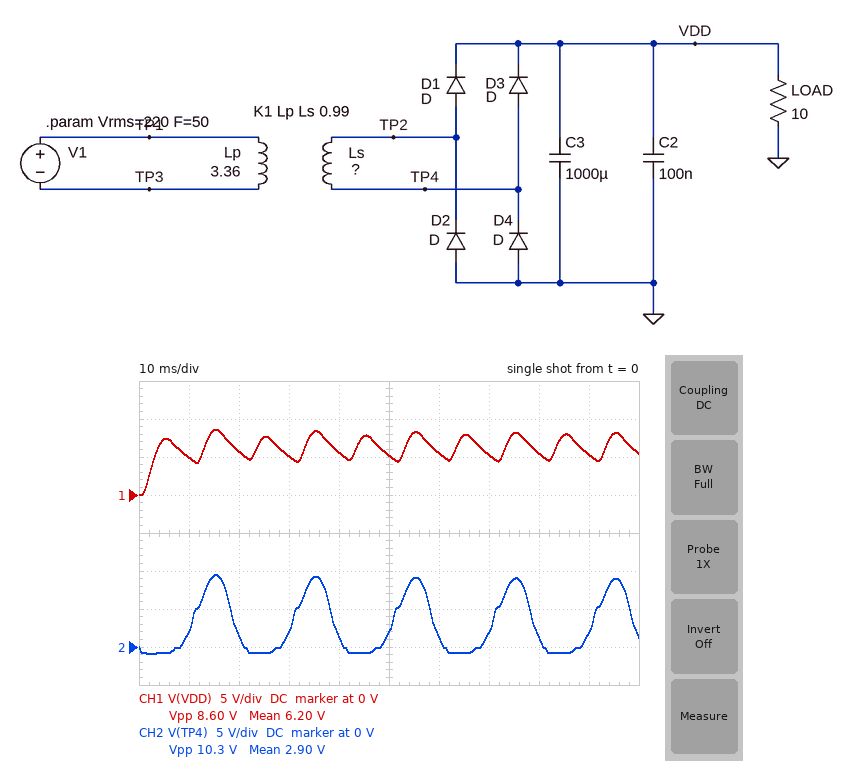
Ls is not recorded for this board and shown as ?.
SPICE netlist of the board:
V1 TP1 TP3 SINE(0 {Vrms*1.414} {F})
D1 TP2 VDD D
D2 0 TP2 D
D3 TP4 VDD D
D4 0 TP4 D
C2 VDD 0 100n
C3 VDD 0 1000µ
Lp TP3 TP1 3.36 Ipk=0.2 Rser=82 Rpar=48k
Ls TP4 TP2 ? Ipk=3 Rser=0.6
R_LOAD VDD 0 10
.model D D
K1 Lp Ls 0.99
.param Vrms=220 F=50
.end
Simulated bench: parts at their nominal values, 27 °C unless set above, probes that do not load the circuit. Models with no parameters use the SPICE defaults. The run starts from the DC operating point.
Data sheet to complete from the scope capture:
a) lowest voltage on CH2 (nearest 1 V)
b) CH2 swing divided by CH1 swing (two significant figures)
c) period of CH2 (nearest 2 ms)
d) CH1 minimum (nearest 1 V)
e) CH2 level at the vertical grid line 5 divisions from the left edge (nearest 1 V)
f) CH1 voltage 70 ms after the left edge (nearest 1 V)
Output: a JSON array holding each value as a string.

["-1 V", "1.2", "20 ms", "0 V", "2 V", "5 V"]
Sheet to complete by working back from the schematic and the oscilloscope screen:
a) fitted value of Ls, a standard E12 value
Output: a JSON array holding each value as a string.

["3.9 mH"]
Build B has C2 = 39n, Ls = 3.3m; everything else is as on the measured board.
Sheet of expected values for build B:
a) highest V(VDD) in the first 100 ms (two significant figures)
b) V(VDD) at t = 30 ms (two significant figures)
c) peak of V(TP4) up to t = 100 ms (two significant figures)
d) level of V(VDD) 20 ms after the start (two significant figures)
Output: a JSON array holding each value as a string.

["7.8 V", "4.6 V", "8.6 V", "5.2 V"]
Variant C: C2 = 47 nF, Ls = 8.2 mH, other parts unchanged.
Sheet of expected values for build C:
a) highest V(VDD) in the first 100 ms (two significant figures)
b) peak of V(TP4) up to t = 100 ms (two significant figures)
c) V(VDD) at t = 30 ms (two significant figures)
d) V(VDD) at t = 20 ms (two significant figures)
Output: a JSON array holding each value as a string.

["13 V", "14 V", "7.8 V", "8.7 V"]
